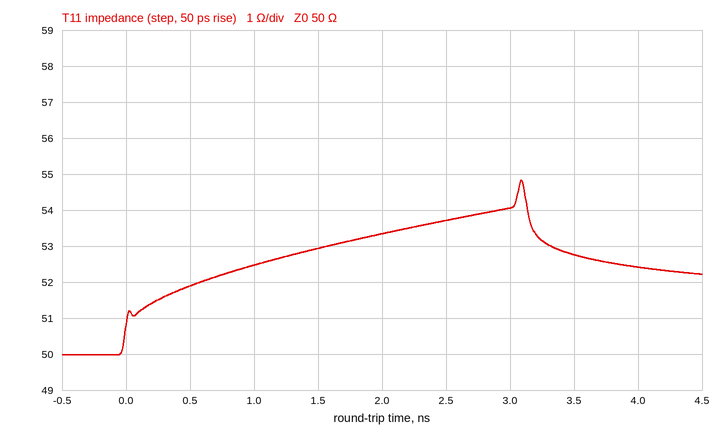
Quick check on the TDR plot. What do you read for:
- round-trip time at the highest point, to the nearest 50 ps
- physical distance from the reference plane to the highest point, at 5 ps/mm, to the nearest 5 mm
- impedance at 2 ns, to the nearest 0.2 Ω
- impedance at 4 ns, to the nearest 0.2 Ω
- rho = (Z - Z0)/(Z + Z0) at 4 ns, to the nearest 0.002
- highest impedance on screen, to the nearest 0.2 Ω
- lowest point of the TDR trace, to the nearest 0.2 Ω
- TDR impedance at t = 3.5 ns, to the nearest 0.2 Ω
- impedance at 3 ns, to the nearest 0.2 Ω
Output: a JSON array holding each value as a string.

["3.10 ns", "310 mm", "53.4 Ω", "52.4 Ω", "+0.024", "54.8 Ω", "50.0 Ω", "52.8 Ω", "54.0 Ω"]
